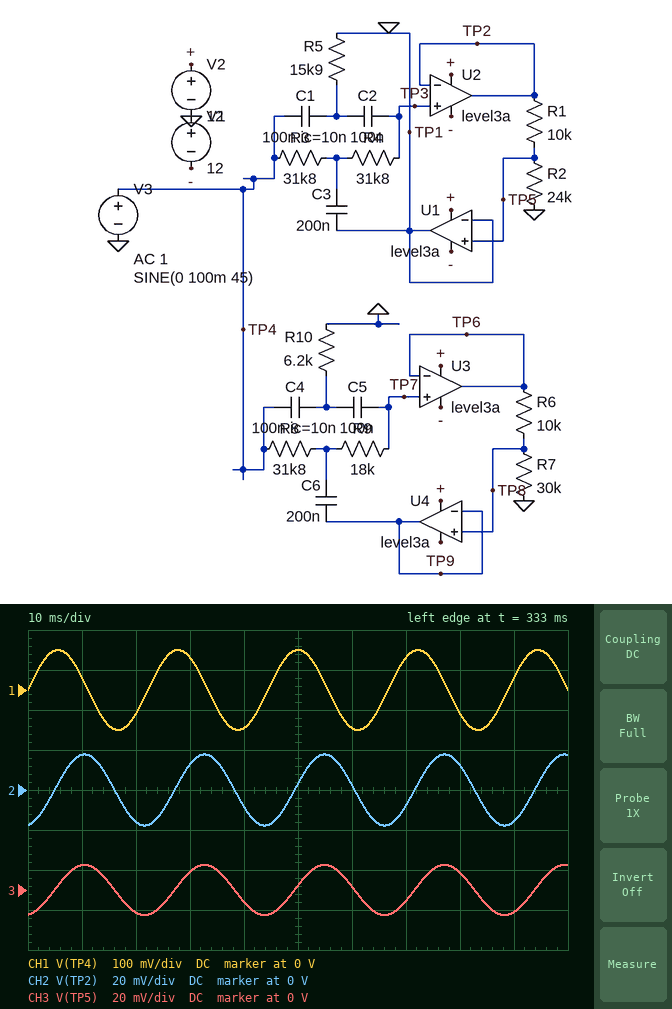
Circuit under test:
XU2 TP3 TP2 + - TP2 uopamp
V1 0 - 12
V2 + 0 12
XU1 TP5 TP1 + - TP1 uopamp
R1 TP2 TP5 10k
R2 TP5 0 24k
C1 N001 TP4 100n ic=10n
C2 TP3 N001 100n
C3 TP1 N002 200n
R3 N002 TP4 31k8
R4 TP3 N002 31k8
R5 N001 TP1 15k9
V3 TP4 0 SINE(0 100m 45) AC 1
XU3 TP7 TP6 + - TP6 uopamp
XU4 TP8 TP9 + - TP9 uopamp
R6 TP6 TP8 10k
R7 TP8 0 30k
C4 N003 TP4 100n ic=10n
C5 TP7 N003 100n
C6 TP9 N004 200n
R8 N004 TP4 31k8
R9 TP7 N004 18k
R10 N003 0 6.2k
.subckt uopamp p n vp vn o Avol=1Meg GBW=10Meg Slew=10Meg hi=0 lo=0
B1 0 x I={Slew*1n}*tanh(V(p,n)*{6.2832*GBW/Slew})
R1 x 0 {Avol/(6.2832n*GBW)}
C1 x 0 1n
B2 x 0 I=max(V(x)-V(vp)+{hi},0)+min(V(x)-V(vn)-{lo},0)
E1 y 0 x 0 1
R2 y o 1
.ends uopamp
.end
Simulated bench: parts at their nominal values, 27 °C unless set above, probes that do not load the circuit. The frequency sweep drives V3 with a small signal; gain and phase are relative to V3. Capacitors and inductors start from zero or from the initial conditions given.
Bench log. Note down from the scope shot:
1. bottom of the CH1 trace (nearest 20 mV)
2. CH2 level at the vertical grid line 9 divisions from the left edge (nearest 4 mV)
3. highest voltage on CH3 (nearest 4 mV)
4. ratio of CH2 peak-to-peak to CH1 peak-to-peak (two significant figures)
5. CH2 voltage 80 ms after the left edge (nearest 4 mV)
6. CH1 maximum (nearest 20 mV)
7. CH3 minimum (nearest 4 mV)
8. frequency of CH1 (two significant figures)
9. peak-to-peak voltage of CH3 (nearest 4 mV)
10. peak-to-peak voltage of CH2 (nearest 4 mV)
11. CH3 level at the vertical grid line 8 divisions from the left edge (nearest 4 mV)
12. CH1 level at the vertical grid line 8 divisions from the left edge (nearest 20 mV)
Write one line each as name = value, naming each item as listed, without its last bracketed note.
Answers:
bottom of the CH1 trace = -100 mV
CH2 level at the vertical grid line 9 divisions from the left edge = -16 mV
highest voltage on CH3 = 12 mV
ratio of CH2 peak-to-peak to CH1 peak-to-peak = 0.18
CH2 voltage 80 ms after the left edge = 12 mV
CH1 maximum = 100 mV
CH3 minimum = -12 mV
frequency of CH1 = 45 Hz
peak-to-peak voltage of CH3 = 24 mV
peak-to-peak voltage of CH2 = 36 mV
CH3 level at the vertical grid line 8 divisions from the left edge = 8 mV
CH1 level at the vertical grid line 8 divisions from the left edge = -60 mV
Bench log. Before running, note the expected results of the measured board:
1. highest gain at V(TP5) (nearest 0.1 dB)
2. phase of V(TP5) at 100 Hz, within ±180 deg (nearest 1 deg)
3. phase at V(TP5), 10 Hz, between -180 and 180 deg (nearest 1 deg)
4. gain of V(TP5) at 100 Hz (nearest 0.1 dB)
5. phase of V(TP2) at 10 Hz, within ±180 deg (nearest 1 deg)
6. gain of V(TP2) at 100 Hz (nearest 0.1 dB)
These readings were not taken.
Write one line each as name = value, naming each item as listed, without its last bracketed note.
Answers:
highest gain at V(TP5) = -3.0 dB
phase of V(TP5) at 100 Hz, within ±180 deg = 38 deg
phase at V(TP5), 10 Hz, between -180 and 180 deg = -14 deg
gain of V(TP5) at 100 Hz = -5.1 dB
phase of V(TP2) at 10 Hz, within ±180 deg = -14 deg
gain of V(TP2) at 100 Hz = -2.1 dB
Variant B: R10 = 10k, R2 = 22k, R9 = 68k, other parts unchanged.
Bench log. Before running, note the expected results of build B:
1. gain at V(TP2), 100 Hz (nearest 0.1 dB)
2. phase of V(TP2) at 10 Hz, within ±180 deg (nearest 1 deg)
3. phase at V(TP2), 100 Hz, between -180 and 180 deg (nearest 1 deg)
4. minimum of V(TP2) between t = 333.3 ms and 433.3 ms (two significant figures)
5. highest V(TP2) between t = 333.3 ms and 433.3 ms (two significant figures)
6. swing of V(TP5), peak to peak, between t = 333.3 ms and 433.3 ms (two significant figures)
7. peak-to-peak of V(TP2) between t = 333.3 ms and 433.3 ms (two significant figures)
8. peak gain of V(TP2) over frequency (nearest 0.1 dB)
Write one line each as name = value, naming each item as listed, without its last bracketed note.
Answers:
gain at V(TP2), 100 Hz = -2.3 dB
phase of V(TP2) at 10 Hz, within ±180 deg = -15 deg
phase at V(TP2), 100 Hz, between -180 and 180 deg = 40 deg
minimum of V(TP2) between t = 333.3 ms and 433.3 ms = -17 mV
highest V(TP2) between t = 333.3 ms and 433.3 ms = 17 mV
swing of V(TP5), peak to peak, between t = 333.3 ms and 433.3 ms = 23 mV
peak-to-peak of V(TP2) between t = 333.3 ms and 433.3 ms = 34 mV
peak gain of V(TP2) over frequency = 0 dB
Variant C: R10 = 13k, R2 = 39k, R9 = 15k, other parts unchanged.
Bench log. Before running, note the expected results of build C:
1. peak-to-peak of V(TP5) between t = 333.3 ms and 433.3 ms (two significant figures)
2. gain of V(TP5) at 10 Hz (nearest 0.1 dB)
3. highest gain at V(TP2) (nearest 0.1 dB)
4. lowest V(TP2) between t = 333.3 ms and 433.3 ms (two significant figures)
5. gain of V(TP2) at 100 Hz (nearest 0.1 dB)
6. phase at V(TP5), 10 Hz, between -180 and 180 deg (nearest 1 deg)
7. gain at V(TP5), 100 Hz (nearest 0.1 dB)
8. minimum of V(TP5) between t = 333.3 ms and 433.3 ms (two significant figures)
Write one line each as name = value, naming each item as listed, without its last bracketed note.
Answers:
peak-to-peak of V(TP5) between t = 333.3 ms and 433.3 ms = 40 mV
gain of V(TP5) at 10 Hz = -2.1 dB
highest gain at V(TP2) = 0 dB
lowest V(TP2) between t = 333.3 ms and 433.3 ms = -25 mV
gain of V(TP2) at 100 Hz = -1.1 dB
phase at V(TP5), 10 Hz, between -180 and 180 deg = -10 deg
gain at V(TP5), 100 Hz = -3.1 dB
minimum of V(TP5) between t = 333.3 ms and 433.3 ms = -20 mV
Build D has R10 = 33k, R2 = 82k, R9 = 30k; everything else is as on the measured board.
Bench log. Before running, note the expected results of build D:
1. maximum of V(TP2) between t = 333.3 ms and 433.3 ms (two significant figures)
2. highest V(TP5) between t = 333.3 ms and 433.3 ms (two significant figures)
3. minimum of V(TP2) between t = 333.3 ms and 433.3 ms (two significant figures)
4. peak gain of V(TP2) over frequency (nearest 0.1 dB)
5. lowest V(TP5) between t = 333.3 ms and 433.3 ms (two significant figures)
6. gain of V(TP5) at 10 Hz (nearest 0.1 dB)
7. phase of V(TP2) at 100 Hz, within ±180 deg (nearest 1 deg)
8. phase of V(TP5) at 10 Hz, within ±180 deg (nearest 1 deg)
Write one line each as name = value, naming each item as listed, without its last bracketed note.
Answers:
maximum of V(TP2) between t = 333.3 ms and 433.3 ms = 44 mV
highest V(TP5) between t = 333.3 ms and 433.3 ms = 39 mV
minimum of V(TP2) between t = 333.3 ms and 433.3 ms = -44 mV
peak gain of V(TP2) over frequency = 0 dB
lowest V(TP5) between t = 333.3 ms and 433.3 ms = -39 mV
gain of V(TP5) at 10 Hz = -1.0 dB
phase of V(TP2) at 100 Hz, within ±180 deg = 16 deg
phase of V(TP5) at 10 Hz, within ±180 deg = -5 deg
